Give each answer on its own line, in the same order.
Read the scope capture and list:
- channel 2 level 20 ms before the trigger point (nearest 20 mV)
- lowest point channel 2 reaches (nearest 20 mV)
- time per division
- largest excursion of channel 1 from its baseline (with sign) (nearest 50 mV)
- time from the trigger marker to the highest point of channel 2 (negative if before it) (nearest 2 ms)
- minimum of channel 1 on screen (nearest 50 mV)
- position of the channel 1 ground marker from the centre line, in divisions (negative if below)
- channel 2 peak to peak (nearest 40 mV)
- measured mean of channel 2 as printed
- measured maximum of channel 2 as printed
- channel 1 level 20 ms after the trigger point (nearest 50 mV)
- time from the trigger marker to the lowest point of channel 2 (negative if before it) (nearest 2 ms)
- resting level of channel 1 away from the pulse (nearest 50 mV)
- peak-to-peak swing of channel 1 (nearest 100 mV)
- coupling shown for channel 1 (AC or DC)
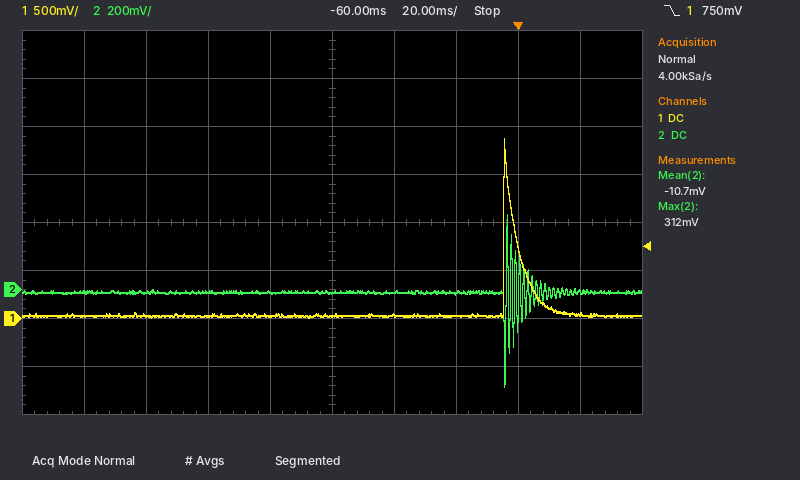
-20 mV
-400 mV
20 ms
+1.85 V
-4 ms
0 mV
-2.0 div
720 mV
-10.7 mV
312 mV
50 mV
-4 ms
50 mV
1.90 V
DC
